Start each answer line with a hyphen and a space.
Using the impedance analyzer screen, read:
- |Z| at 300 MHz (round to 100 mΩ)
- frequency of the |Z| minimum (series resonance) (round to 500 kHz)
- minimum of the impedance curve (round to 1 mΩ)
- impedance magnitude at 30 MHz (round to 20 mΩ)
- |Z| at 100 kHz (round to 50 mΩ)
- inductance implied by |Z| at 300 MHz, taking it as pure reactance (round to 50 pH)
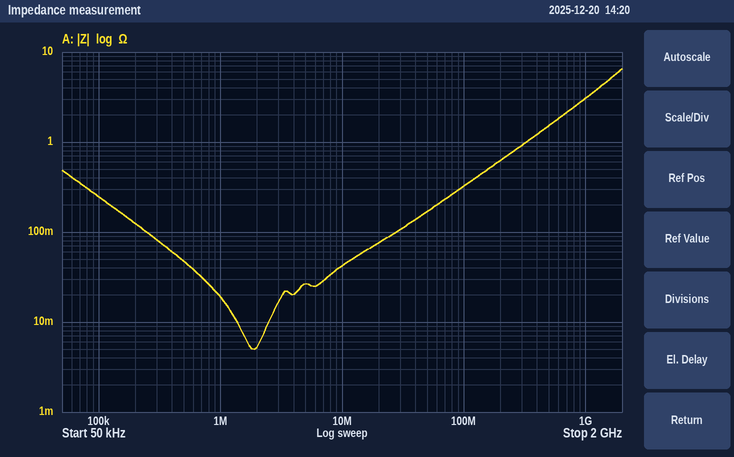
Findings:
- 900 mΩ
- 2.0 MHz
- 5 mΩ
- 100 mΩ
- 250 mΩ
- 500 pH
